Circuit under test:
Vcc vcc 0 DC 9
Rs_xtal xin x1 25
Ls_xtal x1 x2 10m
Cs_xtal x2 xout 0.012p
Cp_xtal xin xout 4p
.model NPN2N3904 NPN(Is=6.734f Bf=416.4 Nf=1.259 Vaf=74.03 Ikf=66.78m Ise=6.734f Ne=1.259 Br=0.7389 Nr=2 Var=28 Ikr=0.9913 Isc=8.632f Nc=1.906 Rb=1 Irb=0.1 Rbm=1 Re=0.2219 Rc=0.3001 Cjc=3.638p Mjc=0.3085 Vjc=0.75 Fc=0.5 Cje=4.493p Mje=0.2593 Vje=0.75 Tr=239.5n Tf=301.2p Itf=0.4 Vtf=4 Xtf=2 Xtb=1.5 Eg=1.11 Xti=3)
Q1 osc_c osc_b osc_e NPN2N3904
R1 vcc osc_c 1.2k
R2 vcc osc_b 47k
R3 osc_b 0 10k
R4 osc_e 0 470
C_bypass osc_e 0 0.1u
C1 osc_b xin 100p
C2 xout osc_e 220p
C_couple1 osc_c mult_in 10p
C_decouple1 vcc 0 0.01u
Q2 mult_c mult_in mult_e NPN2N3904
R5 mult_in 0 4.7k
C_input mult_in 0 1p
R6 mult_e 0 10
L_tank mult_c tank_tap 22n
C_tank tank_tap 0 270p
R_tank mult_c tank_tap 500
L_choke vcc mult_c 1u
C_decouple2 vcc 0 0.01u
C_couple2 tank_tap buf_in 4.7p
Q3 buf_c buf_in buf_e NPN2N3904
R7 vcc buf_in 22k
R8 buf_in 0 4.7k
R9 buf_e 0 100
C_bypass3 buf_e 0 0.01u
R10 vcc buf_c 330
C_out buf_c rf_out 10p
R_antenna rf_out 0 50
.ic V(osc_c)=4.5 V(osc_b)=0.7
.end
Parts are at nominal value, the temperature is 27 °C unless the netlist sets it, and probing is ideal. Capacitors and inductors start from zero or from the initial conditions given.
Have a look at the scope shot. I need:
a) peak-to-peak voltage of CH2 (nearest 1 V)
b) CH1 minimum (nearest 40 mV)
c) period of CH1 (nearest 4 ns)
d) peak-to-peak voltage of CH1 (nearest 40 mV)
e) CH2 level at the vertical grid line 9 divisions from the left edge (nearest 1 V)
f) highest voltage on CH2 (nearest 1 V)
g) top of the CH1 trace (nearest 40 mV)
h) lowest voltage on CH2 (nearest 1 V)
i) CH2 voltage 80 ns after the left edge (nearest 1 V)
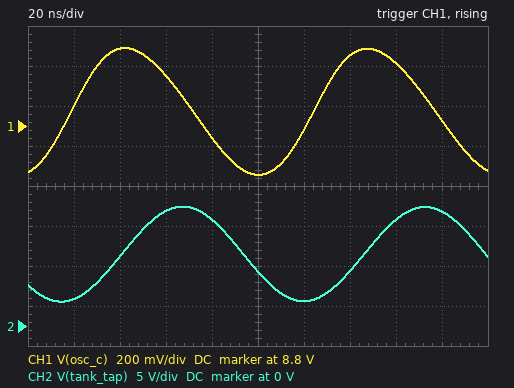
12 V
8.56 V
104 ns
640 mV
14 V
15 V
9.20 V
3 V
13 V
